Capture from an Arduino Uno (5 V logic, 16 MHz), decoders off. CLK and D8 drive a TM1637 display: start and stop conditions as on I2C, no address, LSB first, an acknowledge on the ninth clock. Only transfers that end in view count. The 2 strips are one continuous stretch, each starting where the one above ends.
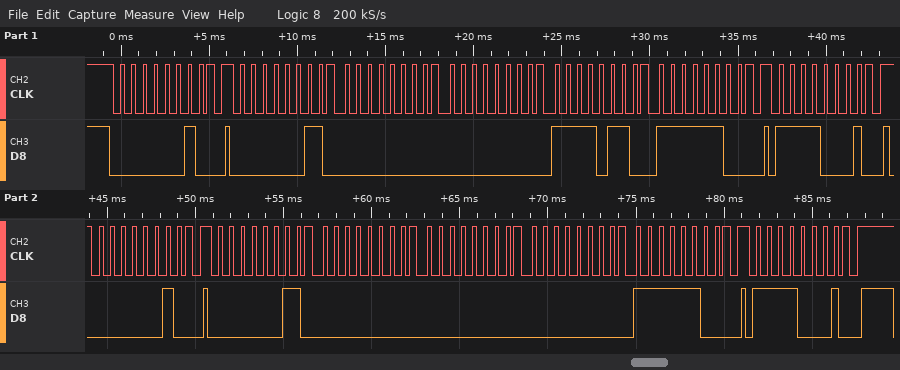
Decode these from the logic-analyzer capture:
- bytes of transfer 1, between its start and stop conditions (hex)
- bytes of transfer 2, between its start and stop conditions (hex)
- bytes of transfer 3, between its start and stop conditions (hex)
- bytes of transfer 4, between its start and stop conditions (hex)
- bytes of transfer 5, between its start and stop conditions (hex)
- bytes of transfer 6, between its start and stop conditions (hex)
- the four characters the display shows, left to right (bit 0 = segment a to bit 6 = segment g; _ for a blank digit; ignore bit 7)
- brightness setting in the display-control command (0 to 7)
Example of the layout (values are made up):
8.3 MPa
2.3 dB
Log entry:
40
C0 00 00 6F 3F
8F
40
C0 00 00 00 3F
8F
___0
7
